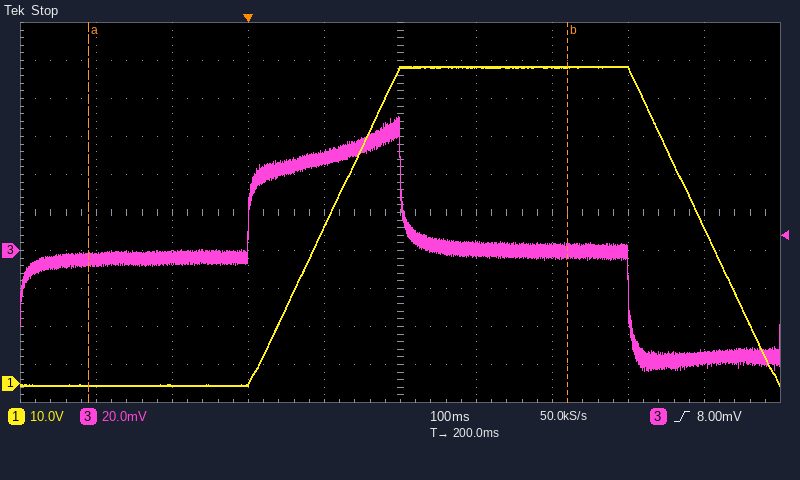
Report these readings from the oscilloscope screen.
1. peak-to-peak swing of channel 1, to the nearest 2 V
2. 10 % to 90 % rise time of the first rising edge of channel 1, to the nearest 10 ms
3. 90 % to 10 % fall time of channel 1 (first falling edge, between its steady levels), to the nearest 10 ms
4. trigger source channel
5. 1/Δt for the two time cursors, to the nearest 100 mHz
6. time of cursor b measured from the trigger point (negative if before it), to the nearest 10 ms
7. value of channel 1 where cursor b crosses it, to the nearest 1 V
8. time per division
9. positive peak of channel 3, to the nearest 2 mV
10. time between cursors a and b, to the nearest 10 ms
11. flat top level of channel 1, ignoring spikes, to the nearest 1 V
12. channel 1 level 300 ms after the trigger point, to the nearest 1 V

84 V
160 ms
160 ms
channel 3
1.6 Hz
+420 ms
83 V
100 ms
70 mV
630 ms
83 V
83 V
